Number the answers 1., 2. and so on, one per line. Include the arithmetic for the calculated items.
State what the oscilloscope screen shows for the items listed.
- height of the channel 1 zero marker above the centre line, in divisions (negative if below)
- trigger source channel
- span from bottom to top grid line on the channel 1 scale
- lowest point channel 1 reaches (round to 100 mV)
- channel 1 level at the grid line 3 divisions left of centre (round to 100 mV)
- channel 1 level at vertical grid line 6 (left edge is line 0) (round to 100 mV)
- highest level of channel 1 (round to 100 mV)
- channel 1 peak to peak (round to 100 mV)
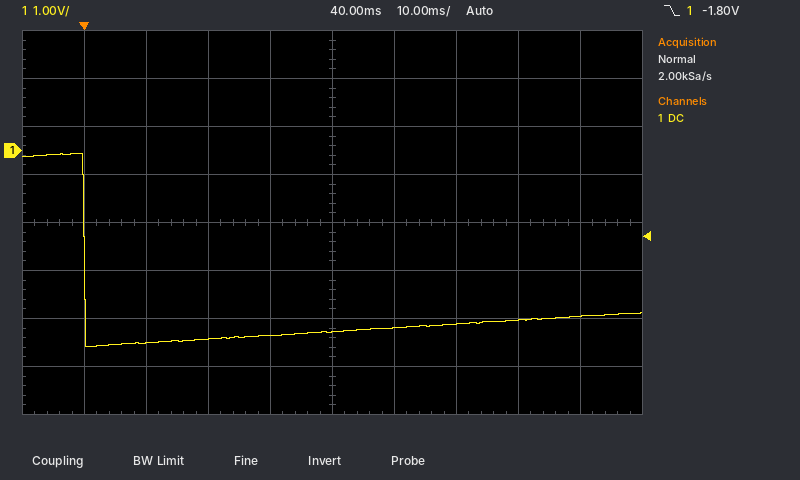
1. +1.5 div
2. channel 1
3. 8 V
4. -4.1 V
5. -4.0 V
6. -3.7 V
7. -100 mV
8. -100 mV − (-4.1 V) = 4.0 V
